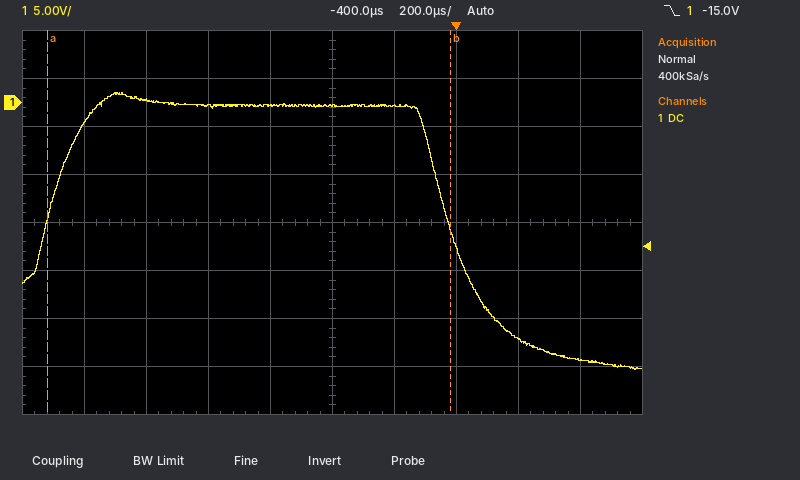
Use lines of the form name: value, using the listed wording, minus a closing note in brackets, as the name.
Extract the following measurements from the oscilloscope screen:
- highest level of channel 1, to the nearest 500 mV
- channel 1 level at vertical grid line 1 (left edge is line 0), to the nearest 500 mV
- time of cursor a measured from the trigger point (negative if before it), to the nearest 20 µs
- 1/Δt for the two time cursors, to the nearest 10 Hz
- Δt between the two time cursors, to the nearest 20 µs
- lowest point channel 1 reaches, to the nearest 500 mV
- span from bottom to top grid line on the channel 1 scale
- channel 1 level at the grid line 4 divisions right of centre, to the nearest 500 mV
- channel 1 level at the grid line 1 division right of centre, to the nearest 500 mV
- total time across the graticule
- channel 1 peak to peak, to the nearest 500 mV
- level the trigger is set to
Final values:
highest level of channel 1, to the nearest 500 mV: 1.0 V
channel 1 level at vertical grid line 1 (left edge is line 0), to the nearest 500 mV: -2.0 V
time of cursor a measured from the trigger point (negative if before it), to the nearest 20 µs: -1.32 ms
1/Δt for the two time cursors, to the nearest 10 Hz: 770 Hz
Δt between the two time cursors, to the nearest 20 µs: 1.30 ms
lowest point channel 1 reaches, to the nearest 500 mV: -28.0 V
span from bottom to top grid line on the channel 1 scale: 40 V
channel 1 level at the grid line 4 divisions right of centre, to the nearest 500 mV: -27.0 V
channel 1 level at the grid line 1 division right of centre, to the nearest 500 mV: -500 mV
total time across the graticule: 2 ms
channel 1 peak to peak, to the nearest 500 mV: 29.0 V
level the trigger is set to: -15.0 V
